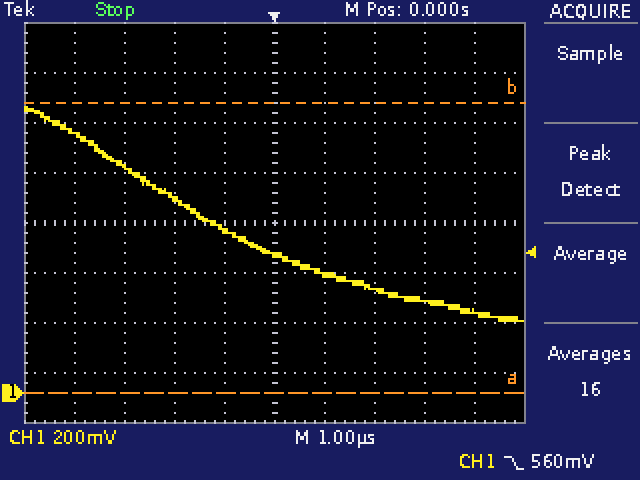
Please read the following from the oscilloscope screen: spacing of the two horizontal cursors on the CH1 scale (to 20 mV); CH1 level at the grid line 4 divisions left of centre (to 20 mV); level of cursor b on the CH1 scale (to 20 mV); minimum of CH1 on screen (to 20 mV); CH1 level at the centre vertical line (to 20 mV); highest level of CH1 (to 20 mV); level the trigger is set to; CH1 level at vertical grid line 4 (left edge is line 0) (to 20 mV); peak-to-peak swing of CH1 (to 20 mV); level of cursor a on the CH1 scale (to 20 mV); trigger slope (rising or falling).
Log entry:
1.16 V
1.04 V
1.16 V
280 mV
560 mV
1.14 V
560 mV
660 mV
860 mV
0 mV
falling
